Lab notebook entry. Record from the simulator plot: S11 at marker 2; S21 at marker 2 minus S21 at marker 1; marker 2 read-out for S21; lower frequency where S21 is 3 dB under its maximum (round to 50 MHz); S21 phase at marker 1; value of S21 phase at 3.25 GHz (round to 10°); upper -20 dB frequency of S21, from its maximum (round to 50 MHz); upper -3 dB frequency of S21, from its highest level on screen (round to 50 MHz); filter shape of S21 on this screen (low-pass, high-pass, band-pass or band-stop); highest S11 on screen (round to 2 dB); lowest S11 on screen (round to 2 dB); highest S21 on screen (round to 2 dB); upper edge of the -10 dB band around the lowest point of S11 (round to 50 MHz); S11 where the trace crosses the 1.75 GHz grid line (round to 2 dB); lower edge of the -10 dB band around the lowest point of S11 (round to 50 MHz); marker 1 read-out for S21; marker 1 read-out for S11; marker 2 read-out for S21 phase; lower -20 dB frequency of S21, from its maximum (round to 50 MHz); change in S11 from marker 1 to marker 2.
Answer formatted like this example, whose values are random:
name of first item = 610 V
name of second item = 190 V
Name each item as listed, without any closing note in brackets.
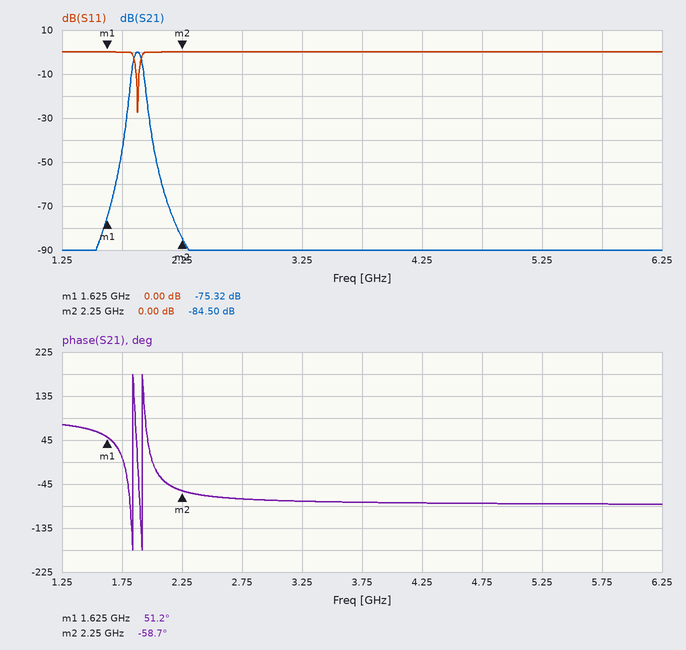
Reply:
S11 at marker 2 = 0.00 dB
S21 at marker 2 minus S21 at marker 1 = -9.18 dB
marker 2 read-out for S21 = -84.50 dB
lower frequency where S21 is 3 dB under its maximum = 1.85 GHz
S21 phase at marker 1 = 51.2°
value of S21 phase at 3.25 GHz = -80°
upper -20 dB frequency of S21, from its maximum = 1.95 GHz
upper -3 dB frequency of S21, from its highest level on screen = 1.90 GHz
filter shape of S21 on this screen = band-pass
highest S11 on screen = 0 dB
lowest S11 on screen = -28 dB
highest S21 on screen = 0 dB
upper edge of the -10 dB band around the lowest point of S11 = 1.90 GHz
S11 where the trace crosses the 1.75 GHz grid line = 0 dB
lower edge of the -10 dB band around the lowest point of S11 = 1.85 GHz
marker 1 read-out for S21 = -75.32 dB
marker 1 read-out for S11 = 0.00 dB
marker 2 read-out for S21 phase = -58.7°
lower -20 dB frequency of S21, from its maximum = 1.80 GHz
change in S11 from marker 1 to marker 2 = 0.00 dB
